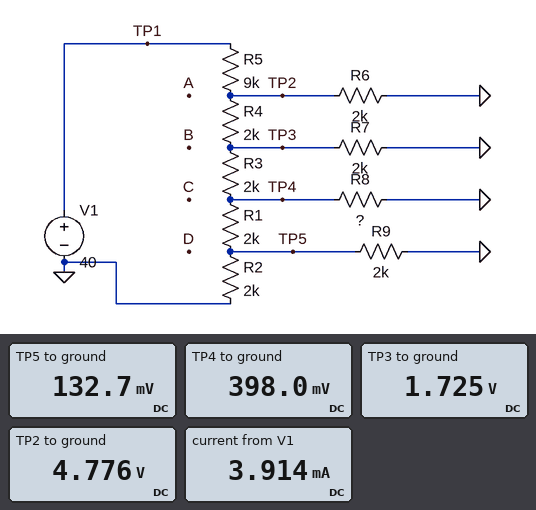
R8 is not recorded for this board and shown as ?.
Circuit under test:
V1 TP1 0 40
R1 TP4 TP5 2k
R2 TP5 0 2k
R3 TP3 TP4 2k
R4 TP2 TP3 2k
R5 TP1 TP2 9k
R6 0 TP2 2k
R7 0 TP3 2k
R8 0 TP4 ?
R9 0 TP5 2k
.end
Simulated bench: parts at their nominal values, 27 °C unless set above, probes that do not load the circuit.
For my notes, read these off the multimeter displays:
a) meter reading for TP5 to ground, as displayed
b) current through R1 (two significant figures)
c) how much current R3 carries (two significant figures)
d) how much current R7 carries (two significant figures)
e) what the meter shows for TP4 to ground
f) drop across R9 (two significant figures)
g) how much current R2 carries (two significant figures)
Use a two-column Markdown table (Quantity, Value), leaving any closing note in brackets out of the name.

| Quantity | Value |
|---|---|
| meter reading for TP5 to ground, as displayed | 132.7 mV |
| current through R1 | 130 µA |
| how much current R3 carries | 660 µA |
| how much current R7 carries | 860 µA |
| what the meter shows for TP4 to ground | 398.0 mV |
| drop across R9 | 130 mV |
| how much current R2 carries | 66 µA |
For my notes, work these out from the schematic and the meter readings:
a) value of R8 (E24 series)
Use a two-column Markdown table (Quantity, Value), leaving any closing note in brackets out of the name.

| Quantity | Value |
|---|---|
| value of R8 | 750 Ω |
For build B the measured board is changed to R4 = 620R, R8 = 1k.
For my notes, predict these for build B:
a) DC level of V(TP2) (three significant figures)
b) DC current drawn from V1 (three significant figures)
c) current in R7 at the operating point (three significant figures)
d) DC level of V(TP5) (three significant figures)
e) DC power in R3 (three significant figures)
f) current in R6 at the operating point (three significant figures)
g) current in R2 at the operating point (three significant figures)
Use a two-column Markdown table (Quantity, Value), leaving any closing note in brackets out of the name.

| Quantity | Value |
|---|---|
| DC level of V(TP2) | 3.79 V |
| DC current drawn from V1 | 4.02 mA |
| current in R7 at the operating point | 1.23 mA |
| DC level of V(TP5) | 224 mV |
| DC power in R3 | 1.61 mW |
| current in R6 at the operating point | 1.89 mA |
| current in R2 at the operating point | 112 µA |
